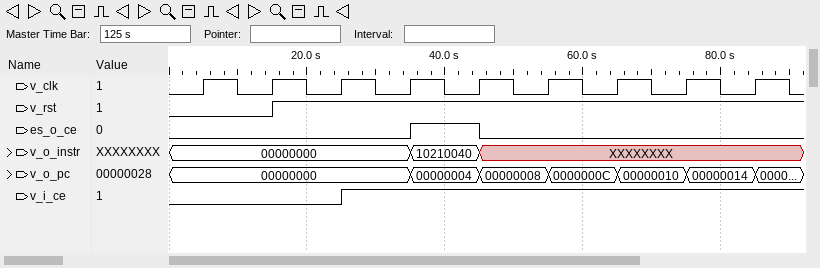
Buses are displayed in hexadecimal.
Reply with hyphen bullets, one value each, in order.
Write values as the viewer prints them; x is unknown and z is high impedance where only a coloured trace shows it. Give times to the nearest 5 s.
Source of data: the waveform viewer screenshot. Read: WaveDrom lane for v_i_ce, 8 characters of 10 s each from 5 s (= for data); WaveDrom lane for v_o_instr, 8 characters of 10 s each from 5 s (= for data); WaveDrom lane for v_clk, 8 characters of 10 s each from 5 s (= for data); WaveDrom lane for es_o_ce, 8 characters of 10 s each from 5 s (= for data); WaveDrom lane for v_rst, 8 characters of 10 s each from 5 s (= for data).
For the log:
- {name: 'v_i_ce', wave: '0.1.....'}
- {name: 'v_o_instr', wave: '=..=x...', data: '00000000 10210040'}
- {name: 'v_clk', wave: 'p.......'}
- {name: 'es_o_ce', wave: '0..10...'}
- {name: 'v_rst', wave: '01......'}
